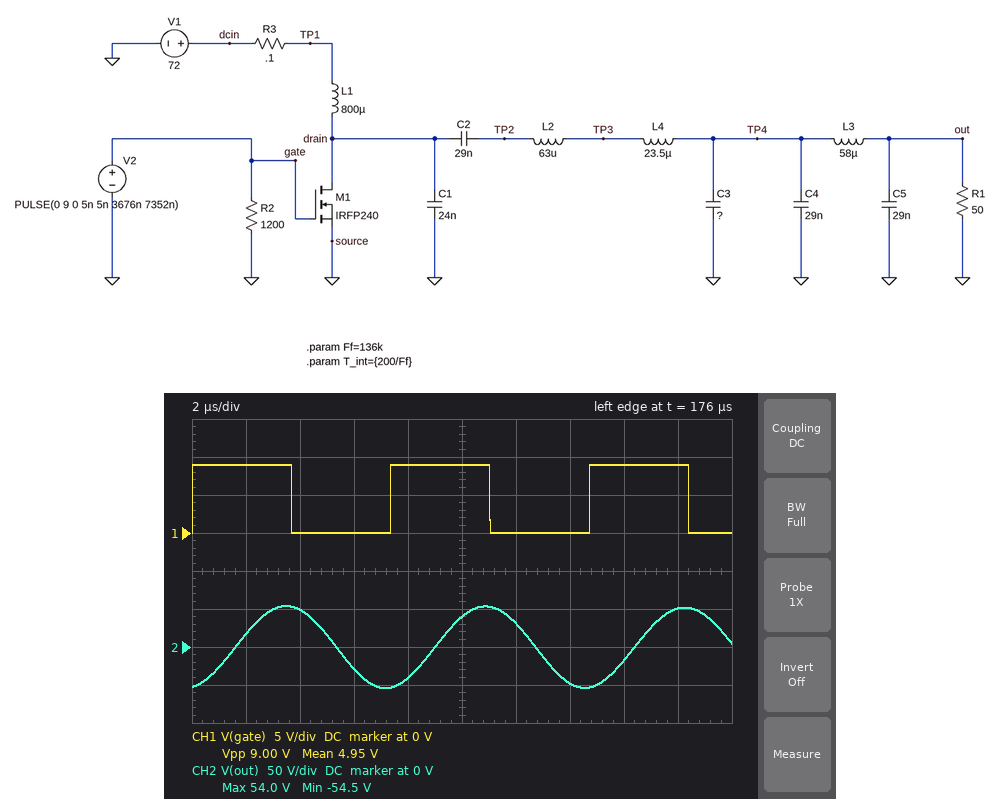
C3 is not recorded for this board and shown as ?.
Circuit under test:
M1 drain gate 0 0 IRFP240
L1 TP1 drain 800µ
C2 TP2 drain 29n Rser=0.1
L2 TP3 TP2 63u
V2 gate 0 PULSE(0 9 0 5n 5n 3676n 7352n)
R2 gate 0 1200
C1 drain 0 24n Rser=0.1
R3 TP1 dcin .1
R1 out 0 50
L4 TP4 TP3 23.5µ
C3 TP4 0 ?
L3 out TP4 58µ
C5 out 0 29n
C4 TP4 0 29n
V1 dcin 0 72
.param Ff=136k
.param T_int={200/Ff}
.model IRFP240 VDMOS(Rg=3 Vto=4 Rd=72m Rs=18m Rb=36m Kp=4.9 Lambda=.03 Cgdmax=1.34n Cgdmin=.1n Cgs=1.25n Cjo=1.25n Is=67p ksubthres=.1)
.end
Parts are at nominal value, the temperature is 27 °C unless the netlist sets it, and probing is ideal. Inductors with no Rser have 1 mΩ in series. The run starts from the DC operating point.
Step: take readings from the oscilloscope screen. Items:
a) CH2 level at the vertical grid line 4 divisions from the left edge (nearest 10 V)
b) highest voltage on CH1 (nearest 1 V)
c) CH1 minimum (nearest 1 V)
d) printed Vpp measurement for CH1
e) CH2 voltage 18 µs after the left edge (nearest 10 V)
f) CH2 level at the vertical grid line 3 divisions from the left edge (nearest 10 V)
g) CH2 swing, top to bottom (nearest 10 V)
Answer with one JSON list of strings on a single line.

["-40 V", "9 V", "0 V", "9.00 V", "50 V", "-30 V", "110 V"]
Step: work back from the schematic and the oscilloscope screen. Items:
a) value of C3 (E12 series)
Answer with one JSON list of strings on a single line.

["120 nF"]
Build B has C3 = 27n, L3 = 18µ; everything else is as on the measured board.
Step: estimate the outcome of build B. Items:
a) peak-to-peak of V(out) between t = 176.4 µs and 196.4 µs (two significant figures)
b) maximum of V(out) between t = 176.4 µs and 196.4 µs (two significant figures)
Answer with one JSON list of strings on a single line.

["180 V", "98 V"]
